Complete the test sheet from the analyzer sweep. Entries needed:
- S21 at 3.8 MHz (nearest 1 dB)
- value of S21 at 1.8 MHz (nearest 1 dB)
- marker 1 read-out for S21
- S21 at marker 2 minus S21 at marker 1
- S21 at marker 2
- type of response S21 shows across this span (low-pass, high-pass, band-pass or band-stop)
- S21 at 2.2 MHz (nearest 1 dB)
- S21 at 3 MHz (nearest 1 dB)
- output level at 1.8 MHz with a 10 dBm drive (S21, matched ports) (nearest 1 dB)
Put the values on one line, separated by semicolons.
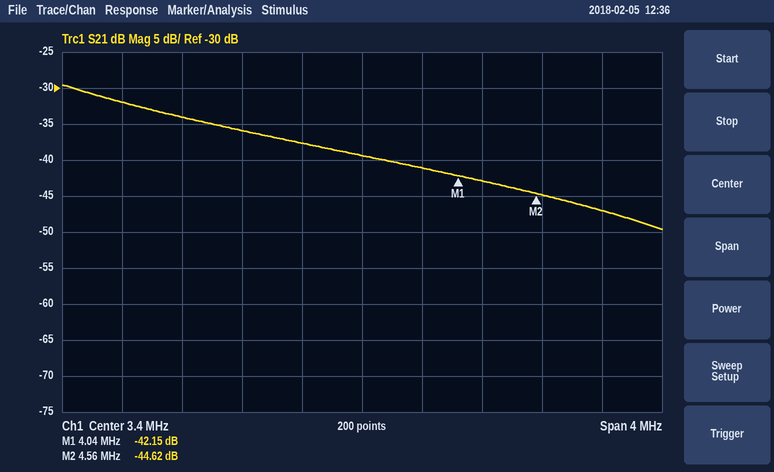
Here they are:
-41 dB; -32 dB; -42.15 dB; -2.47 dB; -44.62 dB; low-pass; -34 dB; -38 dB; -22 dBm
